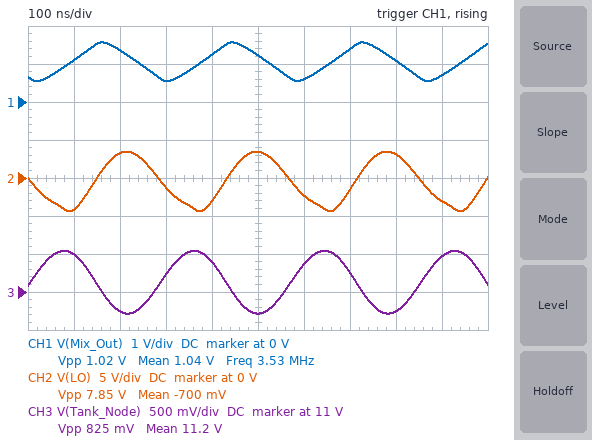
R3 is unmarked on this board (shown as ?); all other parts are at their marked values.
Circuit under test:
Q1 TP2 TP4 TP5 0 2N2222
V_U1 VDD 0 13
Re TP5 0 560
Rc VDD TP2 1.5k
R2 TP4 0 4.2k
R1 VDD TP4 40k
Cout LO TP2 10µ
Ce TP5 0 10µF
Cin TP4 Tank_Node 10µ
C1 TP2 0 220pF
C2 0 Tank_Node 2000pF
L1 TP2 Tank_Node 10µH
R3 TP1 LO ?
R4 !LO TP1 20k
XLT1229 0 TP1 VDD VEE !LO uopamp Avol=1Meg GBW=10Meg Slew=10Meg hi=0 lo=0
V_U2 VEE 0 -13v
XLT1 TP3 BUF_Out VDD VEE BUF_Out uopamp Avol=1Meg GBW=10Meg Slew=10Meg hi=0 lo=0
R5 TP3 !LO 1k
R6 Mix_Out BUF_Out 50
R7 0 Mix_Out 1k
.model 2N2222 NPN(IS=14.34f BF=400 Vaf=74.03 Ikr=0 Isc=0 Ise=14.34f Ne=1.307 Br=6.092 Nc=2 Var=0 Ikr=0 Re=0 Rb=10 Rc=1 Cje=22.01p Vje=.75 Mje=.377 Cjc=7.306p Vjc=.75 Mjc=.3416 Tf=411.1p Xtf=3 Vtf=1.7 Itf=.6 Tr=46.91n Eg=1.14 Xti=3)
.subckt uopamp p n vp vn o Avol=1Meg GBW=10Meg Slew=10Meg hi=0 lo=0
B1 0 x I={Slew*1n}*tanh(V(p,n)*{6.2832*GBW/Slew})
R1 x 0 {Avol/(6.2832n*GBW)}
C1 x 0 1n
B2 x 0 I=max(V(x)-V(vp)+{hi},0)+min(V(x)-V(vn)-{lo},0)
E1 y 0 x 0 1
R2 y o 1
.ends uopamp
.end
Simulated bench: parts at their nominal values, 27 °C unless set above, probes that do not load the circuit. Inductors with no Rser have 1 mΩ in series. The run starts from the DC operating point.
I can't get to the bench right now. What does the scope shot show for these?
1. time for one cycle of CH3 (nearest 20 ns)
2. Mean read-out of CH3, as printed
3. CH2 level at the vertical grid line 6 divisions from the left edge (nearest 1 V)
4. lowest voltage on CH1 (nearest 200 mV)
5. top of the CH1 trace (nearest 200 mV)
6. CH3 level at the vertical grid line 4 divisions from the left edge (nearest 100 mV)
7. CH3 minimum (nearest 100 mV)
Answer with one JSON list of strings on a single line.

["280 ns", "11.2 V", "-2 V", "600 mV", "1.6 V", "11.4 V", "10.7 V"]
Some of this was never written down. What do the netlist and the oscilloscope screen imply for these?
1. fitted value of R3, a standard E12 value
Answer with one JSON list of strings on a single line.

["6.8 kΩ"]
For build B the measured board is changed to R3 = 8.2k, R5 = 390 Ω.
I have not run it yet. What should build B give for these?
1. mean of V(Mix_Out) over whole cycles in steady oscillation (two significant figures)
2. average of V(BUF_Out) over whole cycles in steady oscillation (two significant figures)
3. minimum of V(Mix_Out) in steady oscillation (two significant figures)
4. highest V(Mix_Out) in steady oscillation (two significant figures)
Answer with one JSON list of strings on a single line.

["890 mV", "930 mV", "380 mV", "1.4 V"]
